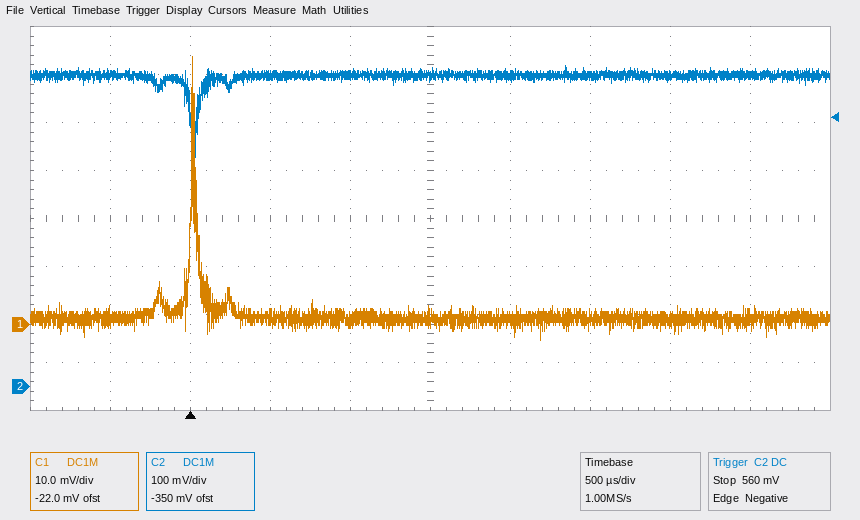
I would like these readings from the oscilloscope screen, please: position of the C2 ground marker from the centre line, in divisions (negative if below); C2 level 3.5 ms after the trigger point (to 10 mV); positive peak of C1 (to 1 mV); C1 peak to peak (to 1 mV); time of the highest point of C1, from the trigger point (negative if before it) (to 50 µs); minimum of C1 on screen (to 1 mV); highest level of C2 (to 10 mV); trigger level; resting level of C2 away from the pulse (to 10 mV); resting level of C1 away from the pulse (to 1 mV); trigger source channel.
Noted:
-3.5 div
650 mV
56 mV
59 mV
0 µs
-3 mV
670 mV
560 mV
650 mV
1 mV
C2
